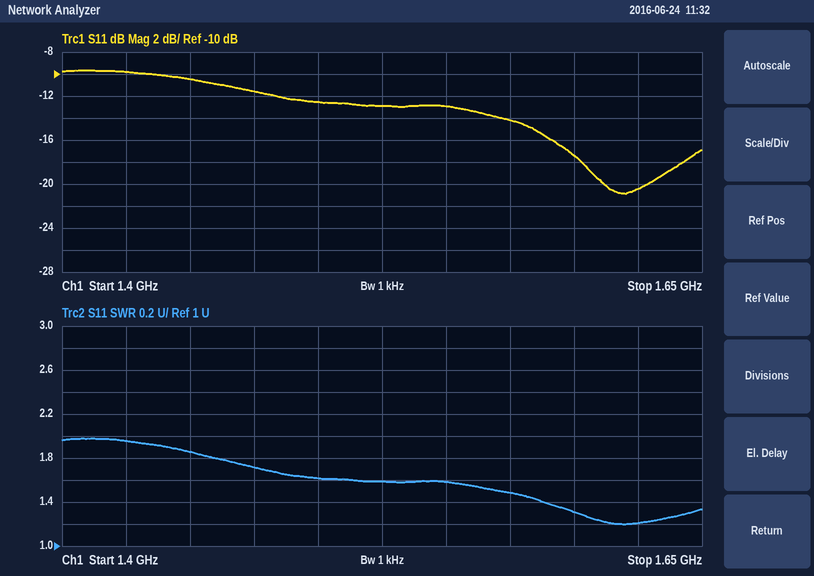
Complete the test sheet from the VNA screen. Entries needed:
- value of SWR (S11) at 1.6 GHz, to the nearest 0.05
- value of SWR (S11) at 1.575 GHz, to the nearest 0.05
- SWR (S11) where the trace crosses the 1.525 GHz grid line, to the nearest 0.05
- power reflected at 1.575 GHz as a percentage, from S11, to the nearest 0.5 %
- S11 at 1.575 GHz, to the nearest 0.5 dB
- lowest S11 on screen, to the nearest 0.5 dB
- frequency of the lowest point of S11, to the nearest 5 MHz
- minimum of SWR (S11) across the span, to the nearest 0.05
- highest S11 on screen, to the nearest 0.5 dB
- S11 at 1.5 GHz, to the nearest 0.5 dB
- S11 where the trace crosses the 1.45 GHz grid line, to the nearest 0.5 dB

1.30
1.50
1.60
4.0 %
-14.0 dB
-21.0 dB
1.620 GHz
1.20
-9.5 dB
-12.5 dB
-10.5 dB
